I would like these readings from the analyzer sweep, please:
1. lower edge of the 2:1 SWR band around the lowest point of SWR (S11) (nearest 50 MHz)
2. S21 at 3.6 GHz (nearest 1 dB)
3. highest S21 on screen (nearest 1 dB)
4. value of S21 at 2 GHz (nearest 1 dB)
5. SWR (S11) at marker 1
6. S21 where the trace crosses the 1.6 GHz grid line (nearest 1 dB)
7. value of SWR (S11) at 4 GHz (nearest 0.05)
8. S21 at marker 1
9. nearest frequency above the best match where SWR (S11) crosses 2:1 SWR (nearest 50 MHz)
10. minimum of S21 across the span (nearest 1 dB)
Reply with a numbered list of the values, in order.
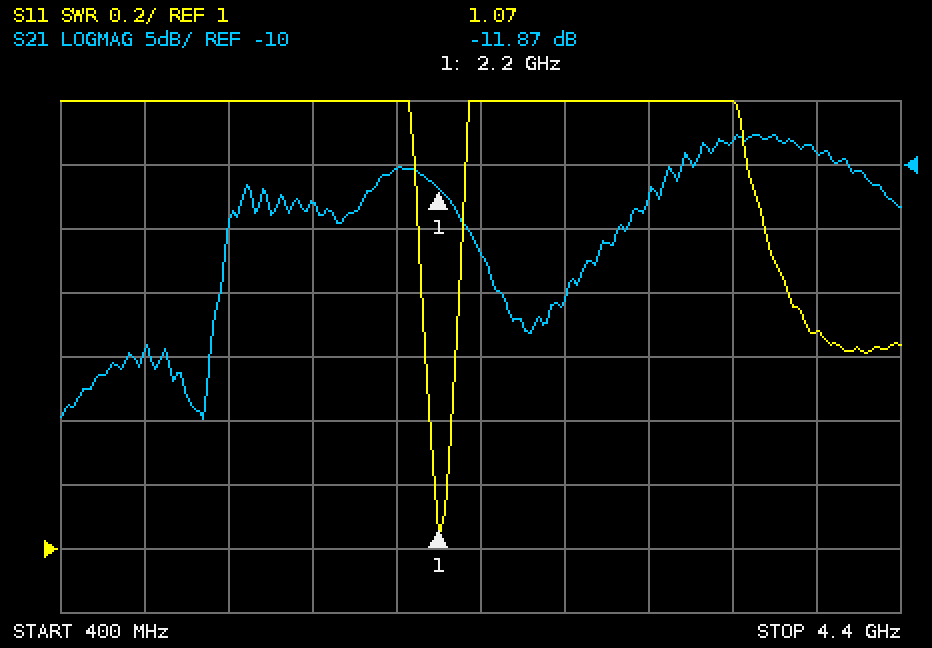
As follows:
1. 2.10 GHz
2. -8 dB
3. -8 dB
4. -10 dB
5. 1.07
6. -13 dB
7. 1.70
8. -11.87 dB
9. 2.30 GHz
10. -30 dB
